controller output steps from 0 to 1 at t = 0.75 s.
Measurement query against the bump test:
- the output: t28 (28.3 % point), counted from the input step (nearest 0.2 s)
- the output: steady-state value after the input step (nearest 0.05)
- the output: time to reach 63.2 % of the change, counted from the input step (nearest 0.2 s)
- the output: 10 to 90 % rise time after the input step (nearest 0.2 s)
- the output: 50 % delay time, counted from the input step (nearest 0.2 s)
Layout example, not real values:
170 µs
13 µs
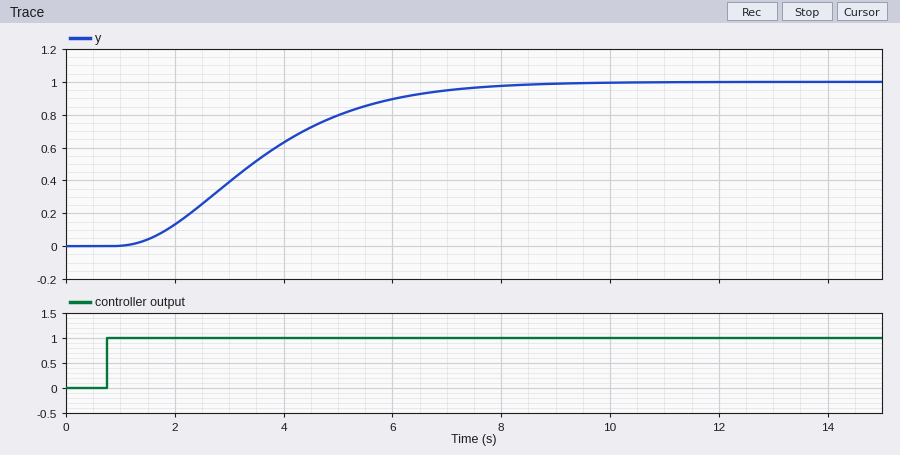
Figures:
1.8 s
1.00
3.2 s
4.2 s
2.6 s
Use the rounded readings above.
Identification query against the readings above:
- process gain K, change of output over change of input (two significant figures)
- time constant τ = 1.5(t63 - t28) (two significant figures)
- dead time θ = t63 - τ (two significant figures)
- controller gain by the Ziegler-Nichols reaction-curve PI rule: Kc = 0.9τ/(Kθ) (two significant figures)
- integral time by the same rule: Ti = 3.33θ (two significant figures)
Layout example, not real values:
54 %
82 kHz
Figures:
1.0
2.1 s
1.1 s
1.7
3.7 s
